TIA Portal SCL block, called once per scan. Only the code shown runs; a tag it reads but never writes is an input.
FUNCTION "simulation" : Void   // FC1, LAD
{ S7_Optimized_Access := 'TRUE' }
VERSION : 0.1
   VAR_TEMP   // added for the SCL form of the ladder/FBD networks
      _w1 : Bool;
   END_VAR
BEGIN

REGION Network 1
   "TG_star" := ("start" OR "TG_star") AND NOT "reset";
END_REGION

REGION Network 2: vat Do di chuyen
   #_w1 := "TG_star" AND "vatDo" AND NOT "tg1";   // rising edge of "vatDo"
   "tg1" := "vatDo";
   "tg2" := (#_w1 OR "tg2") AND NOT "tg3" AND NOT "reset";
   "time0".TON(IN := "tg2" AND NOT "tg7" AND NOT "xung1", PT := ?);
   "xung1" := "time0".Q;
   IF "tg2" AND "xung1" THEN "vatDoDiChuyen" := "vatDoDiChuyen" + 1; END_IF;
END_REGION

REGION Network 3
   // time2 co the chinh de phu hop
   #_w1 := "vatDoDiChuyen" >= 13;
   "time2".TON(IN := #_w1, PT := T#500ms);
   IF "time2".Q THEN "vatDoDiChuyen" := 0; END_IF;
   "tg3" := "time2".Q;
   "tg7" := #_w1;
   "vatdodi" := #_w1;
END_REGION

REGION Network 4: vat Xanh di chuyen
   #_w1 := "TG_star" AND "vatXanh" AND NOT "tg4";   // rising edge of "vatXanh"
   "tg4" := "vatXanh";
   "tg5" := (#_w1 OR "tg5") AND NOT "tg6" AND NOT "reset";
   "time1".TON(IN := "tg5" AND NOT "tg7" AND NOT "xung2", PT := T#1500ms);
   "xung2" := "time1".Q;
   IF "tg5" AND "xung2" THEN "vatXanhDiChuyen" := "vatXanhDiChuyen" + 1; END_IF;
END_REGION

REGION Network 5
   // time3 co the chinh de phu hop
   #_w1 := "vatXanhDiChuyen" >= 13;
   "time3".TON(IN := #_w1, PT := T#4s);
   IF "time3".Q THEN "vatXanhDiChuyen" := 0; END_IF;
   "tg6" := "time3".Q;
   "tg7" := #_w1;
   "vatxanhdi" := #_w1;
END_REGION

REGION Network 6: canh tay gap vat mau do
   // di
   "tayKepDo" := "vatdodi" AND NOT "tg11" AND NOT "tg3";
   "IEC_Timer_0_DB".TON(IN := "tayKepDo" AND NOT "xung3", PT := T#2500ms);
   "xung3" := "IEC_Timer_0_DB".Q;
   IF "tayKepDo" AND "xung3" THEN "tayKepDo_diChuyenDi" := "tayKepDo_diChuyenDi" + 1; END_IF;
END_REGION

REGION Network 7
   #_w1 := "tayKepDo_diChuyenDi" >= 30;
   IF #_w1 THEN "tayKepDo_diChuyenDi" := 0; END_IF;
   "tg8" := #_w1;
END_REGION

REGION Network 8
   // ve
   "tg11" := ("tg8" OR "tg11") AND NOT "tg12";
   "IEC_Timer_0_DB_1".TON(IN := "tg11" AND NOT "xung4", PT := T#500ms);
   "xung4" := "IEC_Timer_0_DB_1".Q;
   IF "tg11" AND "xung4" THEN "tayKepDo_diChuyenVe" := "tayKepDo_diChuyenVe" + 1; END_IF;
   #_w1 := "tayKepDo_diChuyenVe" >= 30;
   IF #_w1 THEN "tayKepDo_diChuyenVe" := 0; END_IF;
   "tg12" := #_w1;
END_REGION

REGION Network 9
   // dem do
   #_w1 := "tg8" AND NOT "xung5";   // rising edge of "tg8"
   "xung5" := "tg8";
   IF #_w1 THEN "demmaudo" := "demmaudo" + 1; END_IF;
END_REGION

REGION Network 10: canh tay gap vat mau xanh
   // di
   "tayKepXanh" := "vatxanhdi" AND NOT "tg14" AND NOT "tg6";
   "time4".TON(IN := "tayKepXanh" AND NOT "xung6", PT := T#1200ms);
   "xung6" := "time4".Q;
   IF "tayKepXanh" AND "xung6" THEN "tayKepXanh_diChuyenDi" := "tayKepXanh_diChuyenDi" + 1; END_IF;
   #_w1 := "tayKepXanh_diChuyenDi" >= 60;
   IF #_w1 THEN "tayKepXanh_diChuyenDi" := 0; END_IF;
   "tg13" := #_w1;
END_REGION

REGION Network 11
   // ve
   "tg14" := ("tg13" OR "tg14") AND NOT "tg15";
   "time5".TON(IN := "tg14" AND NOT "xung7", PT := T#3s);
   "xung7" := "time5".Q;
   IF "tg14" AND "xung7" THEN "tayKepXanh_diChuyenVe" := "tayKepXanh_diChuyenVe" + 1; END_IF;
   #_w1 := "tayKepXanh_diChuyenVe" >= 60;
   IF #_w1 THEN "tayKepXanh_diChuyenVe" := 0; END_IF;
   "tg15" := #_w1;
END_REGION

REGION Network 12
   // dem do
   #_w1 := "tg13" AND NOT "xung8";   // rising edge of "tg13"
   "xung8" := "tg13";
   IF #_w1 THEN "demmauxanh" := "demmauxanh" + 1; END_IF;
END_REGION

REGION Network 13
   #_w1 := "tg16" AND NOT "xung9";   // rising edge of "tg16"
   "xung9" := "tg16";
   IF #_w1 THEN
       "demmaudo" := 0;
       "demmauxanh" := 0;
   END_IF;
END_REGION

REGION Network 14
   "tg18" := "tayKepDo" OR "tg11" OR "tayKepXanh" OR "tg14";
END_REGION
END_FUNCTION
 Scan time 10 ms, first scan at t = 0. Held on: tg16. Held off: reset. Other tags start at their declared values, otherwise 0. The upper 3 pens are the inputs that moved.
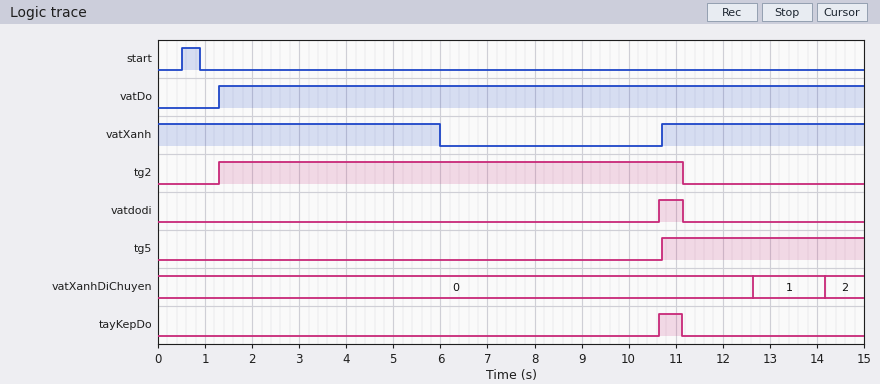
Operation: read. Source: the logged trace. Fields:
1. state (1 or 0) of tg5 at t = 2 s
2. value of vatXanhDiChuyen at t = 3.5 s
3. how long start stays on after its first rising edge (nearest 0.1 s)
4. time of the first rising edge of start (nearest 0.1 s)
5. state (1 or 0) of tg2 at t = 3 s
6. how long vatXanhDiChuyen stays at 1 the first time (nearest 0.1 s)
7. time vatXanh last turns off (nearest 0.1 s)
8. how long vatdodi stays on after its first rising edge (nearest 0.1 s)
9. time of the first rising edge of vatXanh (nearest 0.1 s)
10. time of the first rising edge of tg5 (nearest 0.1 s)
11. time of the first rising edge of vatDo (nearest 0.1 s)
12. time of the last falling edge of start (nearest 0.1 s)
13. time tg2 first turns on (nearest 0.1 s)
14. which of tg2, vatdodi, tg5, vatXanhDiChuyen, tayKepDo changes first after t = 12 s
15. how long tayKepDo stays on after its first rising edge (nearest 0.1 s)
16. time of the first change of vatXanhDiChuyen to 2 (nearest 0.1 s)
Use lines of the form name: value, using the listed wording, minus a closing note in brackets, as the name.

state (1 or 0) of tg5 at t = 2 s: 0
value of vatXanhDiChuyen at t = 3.5 s: 0
how long start stays on after its first rising edge: 0.4 s
time of the first rising edge of start: 0.5 s
state (1 or 0) of tg2 at t = 3 s: 1
how long vatXanhDiChuyen stays at 1 the first time: 1.5 s
time vatXanh last turns off: 6.0 s
how long vatdodi stays on after its first rising edge: 0.5 s
time of the first rising edge of vatXanh: 10.7 s
time of the first rising edge of tg5: 10.7 s
time of the first rising edge of vatDo: 1.3 s
time of the last falling edge of start: 0.9 s
time tg2 first turns on: 1.3 s
which of tg2, vatdodi, tg5, vatXanhDiChuyen, tayKepDo changes first after t = 12 s: vatXanhDiChuyen
how long tayKepDo stays on after its first rising edge: 0.5 s
time of the first change of vatXanhDiChuyen to 2: 14.2 s
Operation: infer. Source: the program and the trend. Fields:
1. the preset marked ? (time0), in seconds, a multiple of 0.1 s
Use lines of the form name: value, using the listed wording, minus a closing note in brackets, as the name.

the preset marked ? (time0), in seconds, a multiple of 0.1 s: 0.7 s
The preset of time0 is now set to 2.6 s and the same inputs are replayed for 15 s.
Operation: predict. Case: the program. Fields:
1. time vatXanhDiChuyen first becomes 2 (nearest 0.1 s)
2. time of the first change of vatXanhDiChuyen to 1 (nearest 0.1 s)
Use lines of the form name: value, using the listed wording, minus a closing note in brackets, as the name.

time vatXanhDiChuyen first becomes 2: 13.7 s
time of the first change of vatXanhDiChuyen to 1: 12.2 s
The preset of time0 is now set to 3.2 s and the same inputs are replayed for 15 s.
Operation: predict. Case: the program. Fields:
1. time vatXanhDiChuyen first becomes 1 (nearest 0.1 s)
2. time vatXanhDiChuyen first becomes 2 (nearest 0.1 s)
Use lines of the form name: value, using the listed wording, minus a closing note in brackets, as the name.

time vatXanhDiChuyen first becomes 1: 12.2 s
time vatXanhDiChuyen first becomes 2: 13.7 s
